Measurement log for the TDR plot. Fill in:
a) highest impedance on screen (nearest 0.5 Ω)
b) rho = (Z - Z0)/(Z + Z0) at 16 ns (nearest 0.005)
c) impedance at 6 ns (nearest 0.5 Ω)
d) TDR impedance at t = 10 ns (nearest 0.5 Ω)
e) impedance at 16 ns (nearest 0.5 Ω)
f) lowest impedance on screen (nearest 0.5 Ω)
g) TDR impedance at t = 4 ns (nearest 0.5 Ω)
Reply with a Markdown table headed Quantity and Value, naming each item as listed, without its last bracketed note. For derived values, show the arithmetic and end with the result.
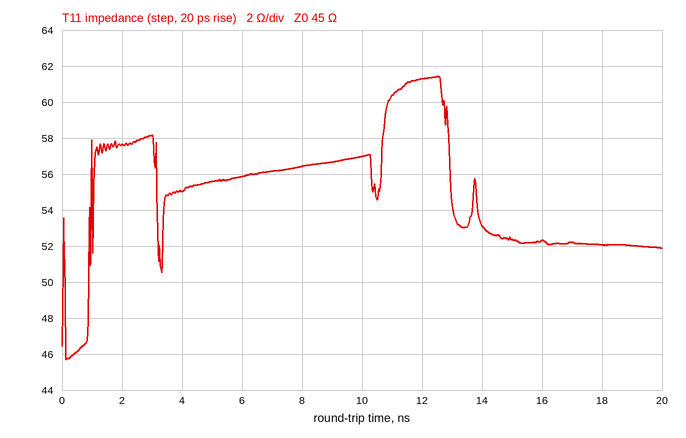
| Quantity | Value |
|---|---|
| highest impedance on screen | 61.5 Ω |
| rho = (Z - Z0)/(Z + Z0) at 16 ns | (52.5 − 45)/(52.5 + 45) ≈ +0.0769, so +0.075 to the nearest 0.005 |
| impedance at 6 ns | 56.0 Ω |
| TDR impedance at t = 10 ns | 57.0 Ω |
| impedance at 16 ns | 52.5 Ω |
| lowest impedance on screen | 45.5 Ω |
| TDR impedance at t = 4 ns | 55.0 Ω |
